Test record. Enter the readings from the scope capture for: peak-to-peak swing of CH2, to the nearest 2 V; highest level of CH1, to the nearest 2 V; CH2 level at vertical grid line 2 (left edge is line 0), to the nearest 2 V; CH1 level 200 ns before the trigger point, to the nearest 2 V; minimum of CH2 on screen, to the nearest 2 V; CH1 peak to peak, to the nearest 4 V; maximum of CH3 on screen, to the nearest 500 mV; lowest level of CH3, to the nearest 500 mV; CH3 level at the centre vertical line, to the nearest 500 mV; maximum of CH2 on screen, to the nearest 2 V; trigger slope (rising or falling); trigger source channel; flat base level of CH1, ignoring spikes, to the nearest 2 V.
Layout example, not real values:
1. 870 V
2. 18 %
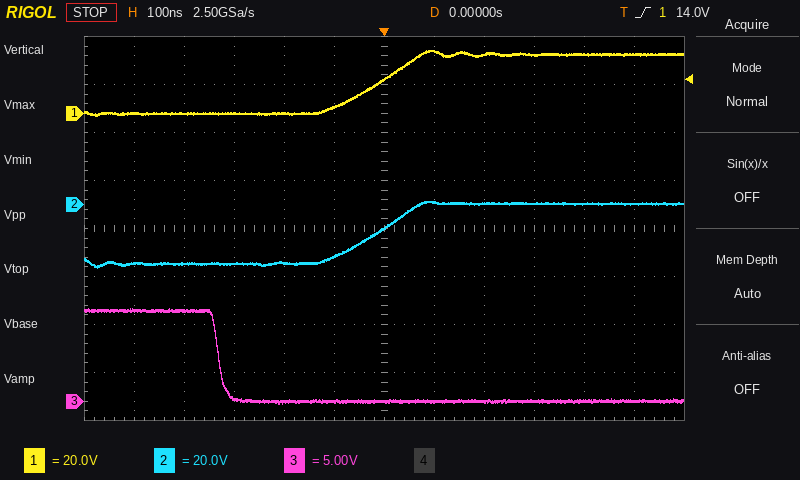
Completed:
1. 28 V
2. 26 V
3. -24 V
4. 0 V
5. -26 V
6. 28 V
7. 9.5 V
8. 0.0 V
9. 0.0 V
10. 2 V
11. rising
12. CH1
13. 0 V
